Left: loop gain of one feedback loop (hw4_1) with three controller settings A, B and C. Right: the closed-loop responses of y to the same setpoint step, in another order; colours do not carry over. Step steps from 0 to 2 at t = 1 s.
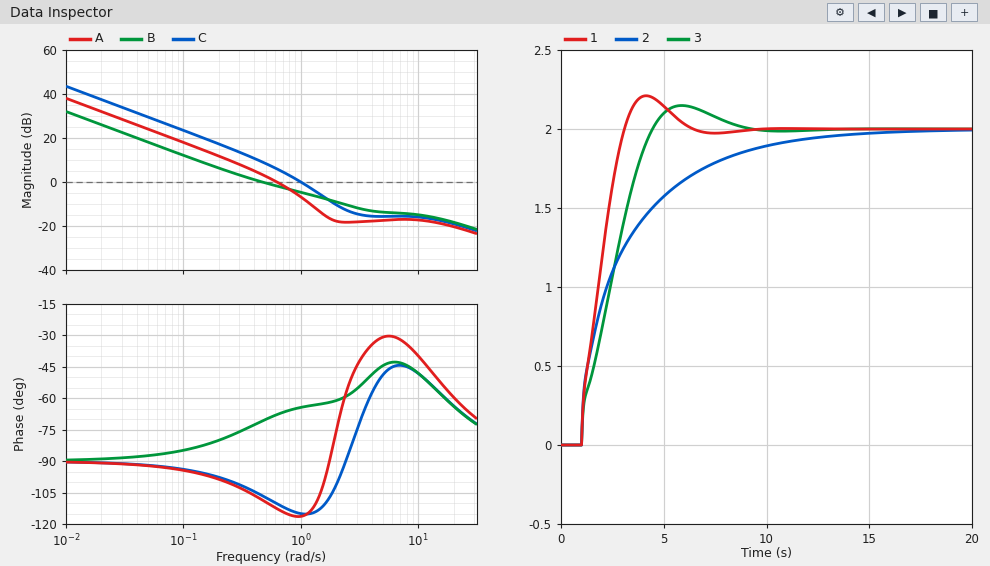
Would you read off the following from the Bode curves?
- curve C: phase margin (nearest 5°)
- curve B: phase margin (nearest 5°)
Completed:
65°
110°
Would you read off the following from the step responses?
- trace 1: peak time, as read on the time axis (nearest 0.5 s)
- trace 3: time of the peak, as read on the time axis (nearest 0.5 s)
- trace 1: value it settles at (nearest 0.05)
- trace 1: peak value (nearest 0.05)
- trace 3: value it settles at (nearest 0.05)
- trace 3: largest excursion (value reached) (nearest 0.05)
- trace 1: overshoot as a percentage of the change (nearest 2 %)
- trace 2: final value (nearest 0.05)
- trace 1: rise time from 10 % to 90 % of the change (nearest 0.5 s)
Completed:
4.0 s
6.0 s
2.00
2.20
2.00
2.15
10 %
2.00
1.5 s
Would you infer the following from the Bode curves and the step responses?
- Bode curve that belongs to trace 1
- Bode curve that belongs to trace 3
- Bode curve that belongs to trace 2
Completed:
C
A
B
